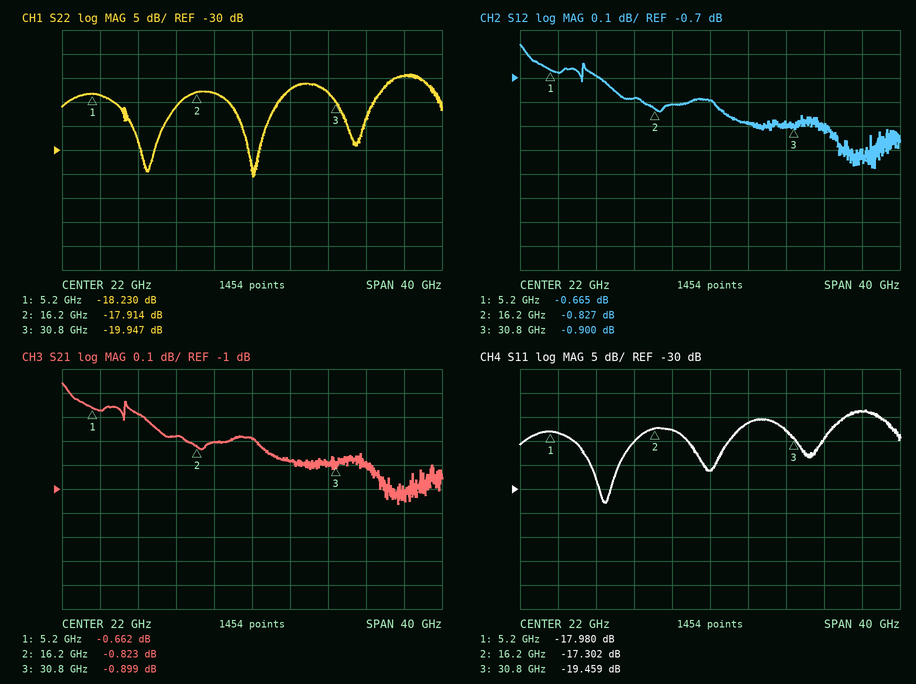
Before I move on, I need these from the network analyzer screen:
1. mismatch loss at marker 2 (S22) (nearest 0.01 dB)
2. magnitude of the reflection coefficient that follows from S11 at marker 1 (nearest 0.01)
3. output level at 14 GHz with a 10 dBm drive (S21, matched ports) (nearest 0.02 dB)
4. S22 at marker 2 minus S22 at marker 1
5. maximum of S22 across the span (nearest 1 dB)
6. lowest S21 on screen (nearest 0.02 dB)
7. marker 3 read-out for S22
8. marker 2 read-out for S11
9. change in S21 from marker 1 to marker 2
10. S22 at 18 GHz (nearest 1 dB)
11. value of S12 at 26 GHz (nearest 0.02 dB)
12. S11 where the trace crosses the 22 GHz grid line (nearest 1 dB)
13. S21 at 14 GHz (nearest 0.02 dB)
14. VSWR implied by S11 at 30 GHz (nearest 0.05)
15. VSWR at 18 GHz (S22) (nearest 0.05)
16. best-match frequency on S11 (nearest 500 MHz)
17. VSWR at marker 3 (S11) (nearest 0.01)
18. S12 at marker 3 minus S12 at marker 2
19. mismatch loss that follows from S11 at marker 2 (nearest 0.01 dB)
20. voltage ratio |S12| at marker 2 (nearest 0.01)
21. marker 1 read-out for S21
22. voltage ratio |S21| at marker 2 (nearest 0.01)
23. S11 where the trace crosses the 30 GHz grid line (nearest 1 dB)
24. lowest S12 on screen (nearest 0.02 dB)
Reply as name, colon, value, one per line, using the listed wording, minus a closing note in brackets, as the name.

mismatch loss at marker 2 (S22): 0.07 dB
magnitude of the reflection coefficient that follows from S11 at marker 1: 0.13
output level at 14 GHz with a 10 dBm drive (S21, matched ports): 9.22 dBm
S22 at marker 2 minus S22 at marker 1: 0.316 dB
maximum of S22 across the span: -14 dB
lowest S21 on screen: -1.06 dB
marker 3 read-out for S22: -19.947 dB
marker 2 read-out for S11: -17.302 dB
change in S21 from marker 1 to marker 2: -0.161 dB
S22 at 18 GHz: -18 dB
value of S12 at 26 GHz: -0.88 dB
S11 where the trace crosses the 22 GHz grid line: -26 dB
S21 at 14 GHz: -0.78 dB
VSWR implied by S11 at 30 GHz: 1.30
VSWR at 18 GHz (S22): 1.30
best-match frequency on S11: 11.0 GHz
VSWR at marker 3 (S11): 1.24
S12 at marker 3 minus S12 at marker 2: -0.073 dB
mismatch loss that follows from S11 at marker 2: 0.08 dB
voltage ratio |S12| at marker 2: 0.91
marker 1 read-out for S21: -0.662 dB
voltage ratio |S21| at marker 2: 0.91
S11 where the trace crosses the 30 GHz grid line: -18 dB
lowest S12 on screen: -1.08 dB
